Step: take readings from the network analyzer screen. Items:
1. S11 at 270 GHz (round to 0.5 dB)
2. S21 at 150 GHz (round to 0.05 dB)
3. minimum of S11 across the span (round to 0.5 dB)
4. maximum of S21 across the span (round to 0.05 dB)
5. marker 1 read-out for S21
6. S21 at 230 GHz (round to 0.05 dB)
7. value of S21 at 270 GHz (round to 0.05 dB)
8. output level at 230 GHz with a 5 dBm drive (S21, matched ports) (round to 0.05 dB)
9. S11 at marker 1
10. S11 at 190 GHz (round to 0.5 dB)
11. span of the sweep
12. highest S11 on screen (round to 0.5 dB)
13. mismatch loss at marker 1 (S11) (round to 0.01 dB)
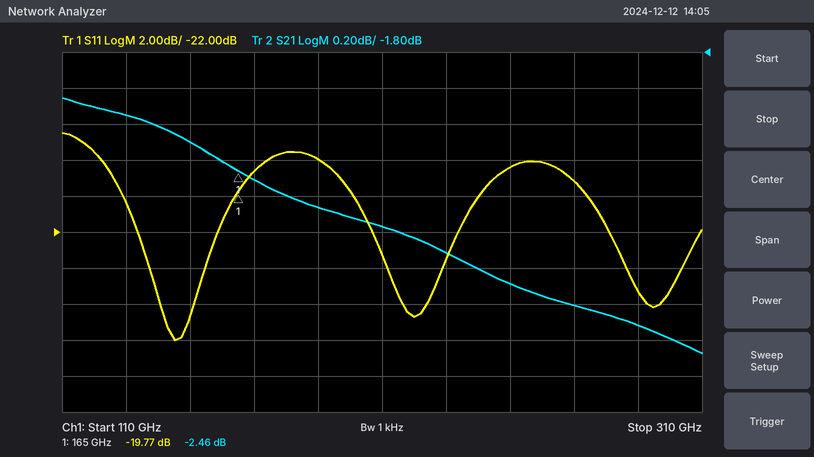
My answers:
-19.0 dB
-2.30 dB
-28.0 dB
-2.05 dB
-2.46 dB
-2.90 dB
-3.20 dB
2.10 dBm
-19.77 dB
-18.0 dB
200 GHz
-16.5 dB
0.05 dB
